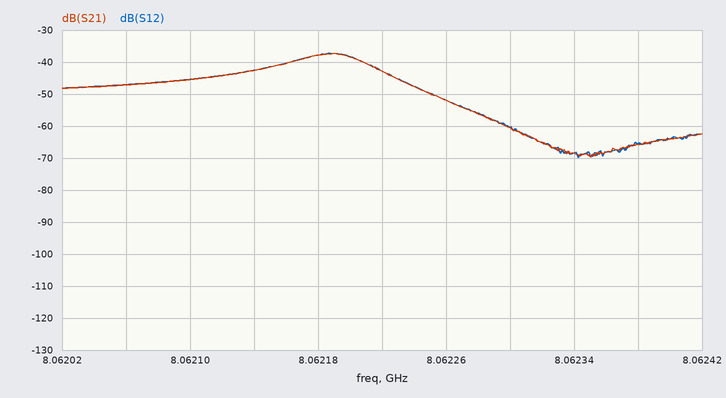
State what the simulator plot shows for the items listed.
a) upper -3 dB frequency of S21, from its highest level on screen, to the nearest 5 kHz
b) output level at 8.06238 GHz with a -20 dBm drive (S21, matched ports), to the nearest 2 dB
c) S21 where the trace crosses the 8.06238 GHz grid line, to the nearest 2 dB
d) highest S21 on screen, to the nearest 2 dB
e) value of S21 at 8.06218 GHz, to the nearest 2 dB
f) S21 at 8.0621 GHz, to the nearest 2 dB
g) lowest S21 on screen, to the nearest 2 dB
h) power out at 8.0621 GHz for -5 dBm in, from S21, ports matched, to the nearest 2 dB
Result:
8.062210 GHz
-86 dBm
-66 dB
-38 dB
-38 dB
-46 dB
-70 dB
-50 dBm
